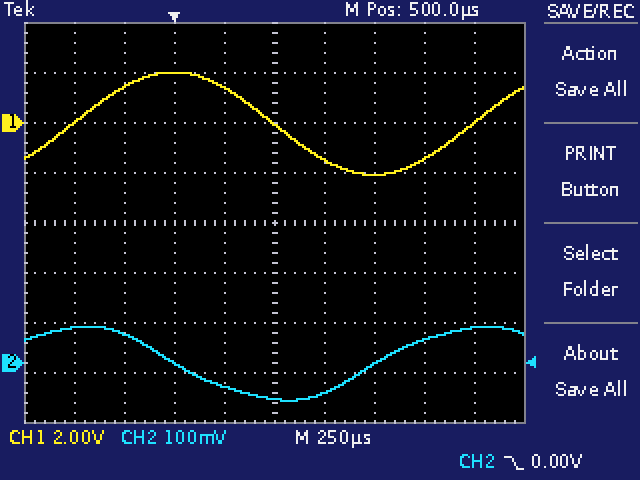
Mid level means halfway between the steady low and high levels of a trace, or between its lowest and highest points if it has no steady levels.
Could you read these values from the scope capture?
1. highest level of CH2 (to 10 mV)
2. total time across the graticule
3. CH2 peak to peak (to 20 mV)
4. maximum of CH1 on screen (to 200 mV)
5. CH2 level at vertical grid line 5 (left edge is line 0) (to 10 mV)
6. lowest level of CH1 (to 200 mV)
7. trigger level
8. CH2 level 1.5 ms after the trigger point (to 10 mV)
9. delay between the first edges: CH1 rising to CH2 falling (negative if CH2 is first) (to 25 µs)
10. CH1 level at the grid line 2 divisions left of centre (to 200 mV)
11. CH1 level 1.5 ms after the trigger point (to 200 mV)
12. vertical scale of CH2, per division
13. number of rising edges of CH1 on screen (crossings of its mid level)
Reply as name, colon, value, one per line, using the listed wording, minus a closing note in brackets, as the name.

highest level of CH2: 70 mV
total time across the graticule: 2.5 ms
CH2 peak to peak: 140 mV
maximum of CH1 on screen: 2.0 V
CH2 level at vertical grid line 5 (left edge is line 0): -70 mV
lowest level of CH1: -2.0 V
trigger level: 0.00 V
CH2 level 1.5 ms after the trigger point: 70 mV
delay between the first edges: CH1 rising to CH2 falling (negative if CH2 is first): +500 µs
CH1 level at the grid line 2 divisions left of centre: 2.0 V
CH1 level 1.5 ms after the trigger point: 0.0 V
vertical scale of CH2, per division: 100 mV
number of rising edges of CH1 on screen: 2
